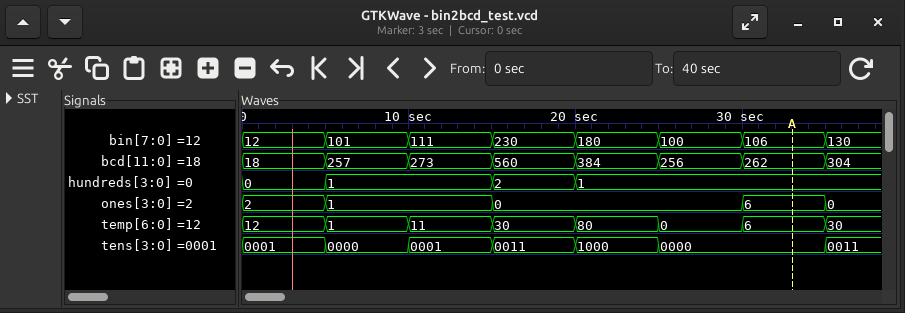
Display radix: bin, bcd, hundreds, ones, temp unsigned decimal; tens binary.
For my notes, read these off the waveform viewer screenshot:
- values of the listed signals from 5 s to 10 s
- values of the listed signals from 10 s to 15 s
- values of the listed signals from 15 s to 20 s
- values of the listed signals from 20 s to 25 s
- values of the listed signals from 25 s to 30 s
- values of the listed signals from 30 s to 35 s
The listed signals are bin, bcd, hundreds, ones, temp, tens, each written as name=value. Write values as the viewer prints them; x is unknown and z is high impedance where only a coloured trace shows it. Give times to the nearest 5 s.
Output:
bin=101, bcd=257, hundreds=1, ones=1, temp=1, tens=0000
bin=111, bcd=273, hundreds=1, ones=1, temp=11, tens=0001
bin=230, bcd=560, hundreds=2, ones=0, temp=30, tens=0011
bin=180, bcd=384, hundreds=1, ones=0, temp=80, tens=1000
bin=100, bcd=256, hundreds=1, ones=0, temp=0, tens=0000
bin=106, bcd=262, hundreds=1, ones=6, temp=6, tens=0000
